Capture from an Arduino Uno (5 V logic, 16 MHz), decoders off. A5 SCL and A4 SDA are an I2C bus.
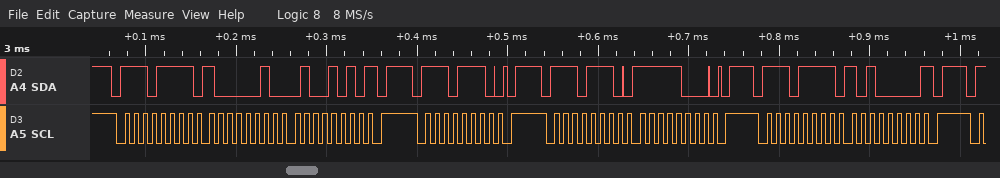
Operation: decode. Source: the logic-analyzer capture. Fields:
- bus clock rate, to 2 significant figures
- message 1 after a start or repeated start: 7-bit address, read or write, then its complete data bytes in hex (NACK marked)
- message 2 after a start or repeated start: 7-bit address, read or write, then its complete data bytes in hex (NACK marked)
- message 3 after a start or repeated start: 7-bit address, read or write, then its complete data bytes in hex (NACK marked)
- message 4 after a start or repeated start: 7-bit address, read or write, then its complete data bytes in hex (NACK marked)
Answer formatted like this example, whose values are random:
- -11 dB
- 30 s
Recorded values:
- 100 kHz
- 0x77 read: 82 4A NACK
- 0x77 write
- 0x77 write: F8
- 0x77 read: A0 NACK
